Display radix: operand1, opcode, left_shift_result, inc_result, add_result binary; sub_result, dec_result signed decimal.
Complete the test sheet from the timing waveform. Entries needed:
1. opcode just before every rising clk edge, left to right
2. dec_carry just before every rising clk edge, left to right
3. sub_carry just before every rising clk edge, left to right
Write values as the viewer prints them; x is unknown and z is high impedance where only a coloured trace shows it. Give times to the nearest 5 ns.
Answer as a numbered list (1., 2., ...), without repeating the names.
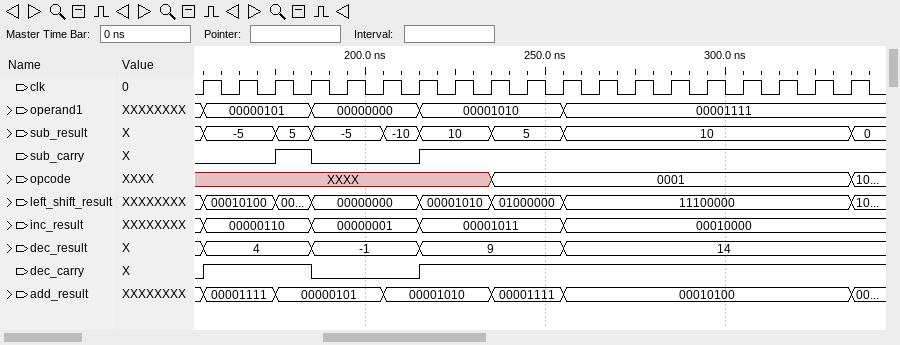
1. XXXX, XXXX, XXXX, XXXX, XXXX, XXXX, XXXX, XXXX, XXXX, 0001, 0001, 0001, 0001, 0001, 0001, 0001, 0001, 0001, 0001
2. 0 1 1 1 0 0 0 1 1 1 1 1 1 1 1 1 1 1 1
3. 0 0 0 1 0 0 0 1 1 1 1 1 1 1 1 1 1 1 1
